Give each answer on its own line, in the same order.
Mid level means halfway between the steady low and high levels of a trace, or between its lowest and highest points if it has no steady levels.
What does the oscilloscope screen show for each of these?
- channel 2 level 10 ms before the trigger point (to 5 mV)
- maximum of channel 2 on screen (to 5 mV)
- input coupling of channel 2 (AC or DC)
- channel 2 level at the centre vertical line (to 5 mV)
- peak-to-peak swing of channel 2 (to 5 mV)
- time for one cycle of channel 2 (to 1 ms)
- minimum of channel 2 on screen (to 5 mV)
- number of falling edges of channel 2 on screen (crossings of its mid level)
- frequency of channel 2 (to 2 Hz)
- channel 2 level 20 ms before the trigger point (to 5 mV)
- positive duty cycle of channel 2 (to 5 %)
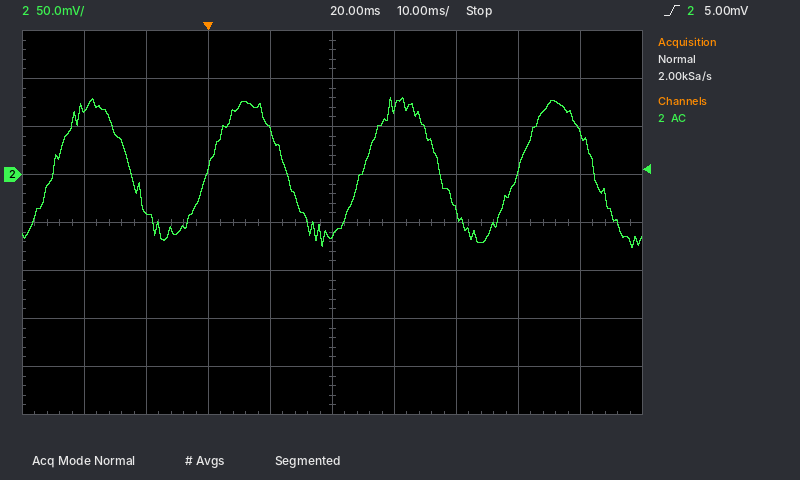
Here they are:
-40 mV
80 mV
AC
-65 mV
155 mV
25 ms
-75 mV
4
40 Hz
70 mV
50 %
